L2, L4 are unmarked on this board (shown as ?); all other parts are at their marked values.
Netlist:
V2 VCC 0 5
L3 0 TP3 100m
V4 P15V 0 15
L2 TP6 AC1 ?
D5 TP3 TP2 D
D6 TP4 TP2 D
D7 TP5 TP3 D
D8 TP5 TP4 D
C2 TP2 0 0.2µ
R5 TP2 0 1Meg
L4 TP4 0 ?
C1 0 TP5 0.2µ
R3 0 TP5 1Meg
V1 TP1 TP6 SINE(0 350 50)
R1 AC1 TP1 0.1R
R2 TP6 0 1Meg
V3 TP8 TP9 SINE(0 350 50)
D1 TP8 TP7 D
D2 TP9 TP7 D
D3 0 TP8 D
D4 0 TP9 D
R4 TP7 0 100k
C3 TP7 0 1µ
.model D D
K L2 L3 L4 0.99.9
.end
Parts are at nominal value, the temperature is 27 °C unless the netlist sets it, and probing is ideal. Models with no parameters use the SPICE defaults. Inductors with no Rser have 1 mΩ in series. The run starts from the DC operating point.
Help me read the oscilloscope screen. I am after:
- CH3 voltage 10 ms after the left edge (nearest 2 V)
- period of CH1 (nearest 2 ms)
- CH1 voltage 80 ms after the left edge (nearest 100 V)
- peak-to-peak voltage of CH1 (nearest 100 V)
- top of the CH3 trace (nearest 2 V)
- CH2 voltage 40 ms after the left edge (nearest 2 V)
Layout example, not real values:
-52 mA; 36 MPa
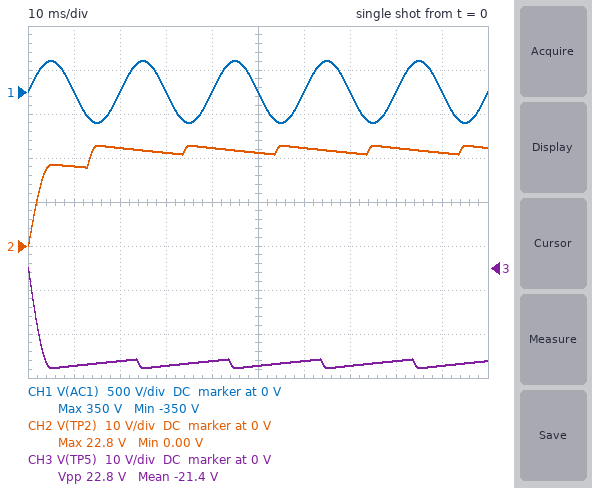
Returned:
-22 V; 20 ms; 0 V; 700 V; 0 V; 22 V
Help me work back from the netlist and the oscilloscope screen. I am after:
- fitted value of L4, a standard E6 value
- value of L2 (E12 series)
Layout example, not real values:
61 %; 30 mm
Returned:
150 mH; 33 H
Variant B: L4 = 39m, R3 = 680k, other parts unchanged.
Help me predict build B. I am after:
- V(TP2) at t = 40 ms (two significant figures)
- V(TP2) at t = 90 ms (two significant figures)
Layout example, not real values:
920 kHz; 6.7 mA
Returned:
17 V; 18 V
